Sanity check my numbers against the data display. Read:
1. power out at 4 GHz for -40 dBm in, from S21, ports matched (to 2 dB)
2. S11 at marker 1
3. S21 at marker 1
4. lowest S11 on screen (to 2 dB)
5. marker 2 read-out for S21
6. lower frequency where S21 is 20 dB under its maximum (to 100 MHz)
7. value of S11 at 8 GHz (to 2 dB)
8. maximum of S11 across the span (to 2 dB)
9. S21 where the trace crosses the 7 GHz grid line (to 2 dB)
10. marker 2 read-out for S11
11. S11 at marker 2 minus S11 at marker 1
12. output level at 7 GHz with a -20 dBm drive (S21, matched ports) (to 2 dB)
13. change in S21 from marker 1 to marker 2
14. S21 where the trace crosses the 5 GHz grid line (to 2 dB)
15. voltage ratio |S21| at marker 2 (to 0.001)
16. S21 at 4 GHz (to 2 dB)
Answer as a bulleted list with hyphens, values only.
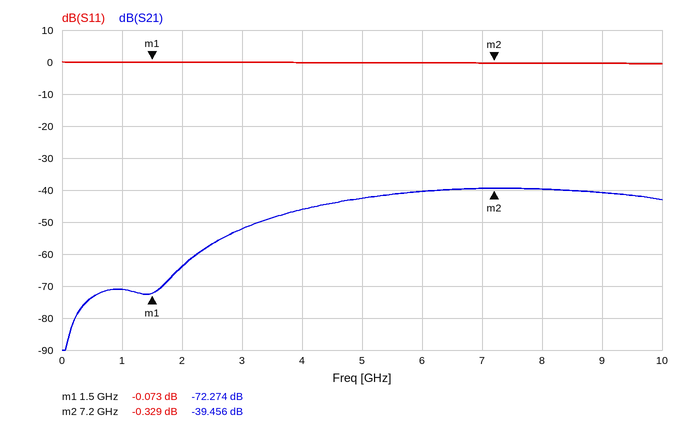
- -86 dBm
- -0.073 dB
- -72.274 dB
- 0 dB
- -39.456 dB
- 2.3 GHz
- 0 dB
- 0 dB
- -40 dB
- -0.329 dB
- -0.256 dB
- -60 dBm
- 32.818 dB
- -42 dB
- 0.011
- -46 dB
